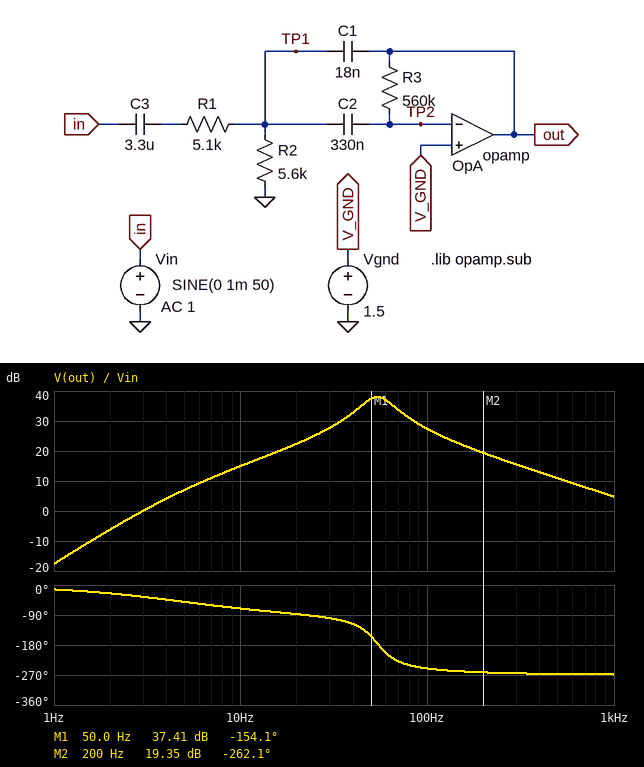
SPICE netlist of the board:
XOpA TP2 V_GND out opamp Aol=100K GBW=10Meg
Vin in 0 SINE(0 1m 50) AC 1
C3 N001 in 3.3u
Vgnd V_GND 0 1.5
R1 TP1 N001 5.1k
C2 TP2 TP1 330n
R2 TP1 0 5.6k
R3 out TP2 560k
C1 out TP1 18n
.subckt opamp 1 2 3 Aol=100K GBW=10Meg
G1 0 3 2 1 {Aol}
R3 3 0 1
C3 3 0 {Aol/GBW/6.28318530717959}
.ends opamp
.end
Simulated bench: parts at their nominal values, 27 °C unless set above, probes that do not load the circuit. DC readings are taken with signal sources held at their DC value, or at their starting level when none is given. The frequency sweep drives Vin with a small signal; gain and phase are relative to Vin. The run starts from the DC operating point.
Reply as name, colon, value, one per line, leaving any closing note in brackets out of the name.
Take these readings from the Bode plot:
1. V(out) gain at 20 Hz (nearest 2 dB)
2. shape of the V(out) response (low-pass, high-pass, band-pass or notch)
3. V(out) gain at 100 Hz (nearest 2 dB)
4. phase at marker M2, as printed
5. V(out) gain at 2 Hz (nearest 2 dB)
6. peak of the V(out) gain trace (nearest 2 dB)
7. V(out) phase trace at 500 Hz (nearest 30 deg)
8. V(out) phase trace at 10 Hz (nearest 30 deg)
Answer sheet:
V(out) gain at 20 Hz: 22 dB
shape of the V(out) response: band-pass
V(out) gain at 100 Hz: 28 dB
phase at marker M2, as printed: -262.1 deg
V(out) gain at 2 Hz: -6 dB
peak of the V(out) gain trace: 38 dB
V(out) phase trace at 500 Hz: -270 deg
V(out) phase trace at 10 Hz: -60 deg
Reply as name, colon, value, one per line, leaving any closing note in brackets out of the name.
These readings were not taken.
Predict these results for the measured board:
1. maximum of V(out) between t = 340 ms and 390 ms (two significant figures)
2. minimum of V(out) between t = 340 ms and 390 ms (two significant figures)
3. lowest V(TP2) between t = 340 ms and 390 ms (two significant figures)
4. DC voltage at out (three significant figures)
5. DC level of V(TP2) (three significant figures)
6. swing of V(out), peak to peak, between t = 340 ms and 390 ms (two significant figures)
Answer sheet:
maximum of V(out) between t = 340 ms and 390 ms: 1.6 V
minimum of V(out) between t = 340 ms and 390 ms: 1.4 V
lowest V(TP2) between t = 340 ms and 390 ms: 1.5 V
DC voltage at out: 1.50 V
DC level of V(TP2): 1.50 V
swing of V(out), peak to peak, between t = 340 ms and 390 ms: 150 mV
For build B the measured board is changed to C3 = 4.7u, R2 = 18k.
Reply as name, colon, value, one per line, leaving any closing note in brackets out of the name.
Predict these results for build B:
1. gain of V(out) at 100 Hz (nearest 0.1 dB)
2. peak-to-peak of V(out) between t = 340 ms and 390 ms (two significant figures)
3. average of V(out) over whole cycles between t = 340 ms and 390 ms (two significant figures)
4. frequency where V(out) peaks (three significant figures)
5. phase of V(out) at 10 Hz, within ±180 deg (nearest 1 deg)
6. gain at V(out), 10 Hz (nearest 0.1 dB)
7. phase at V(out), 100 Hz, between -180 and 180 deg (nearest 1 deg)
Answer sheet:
gain of V(out) at 100 Hz: 26.4 dB
peak-to-peak of V(out) between t = 340 ms and 390 ms: 140 mV
average of V(out) over whole cycles between t = 340 ms and 390 ms: 1.5 V
frequency where V(out) peaks: 44.7 Hz
phase of V(out) at 10 Hz, within ±180 deg: -89 deg
gain at V(out), 10 Hz: 19.1 dB
phase at V(out), 100 Hz, between -180 and 180 deg: 106 deg
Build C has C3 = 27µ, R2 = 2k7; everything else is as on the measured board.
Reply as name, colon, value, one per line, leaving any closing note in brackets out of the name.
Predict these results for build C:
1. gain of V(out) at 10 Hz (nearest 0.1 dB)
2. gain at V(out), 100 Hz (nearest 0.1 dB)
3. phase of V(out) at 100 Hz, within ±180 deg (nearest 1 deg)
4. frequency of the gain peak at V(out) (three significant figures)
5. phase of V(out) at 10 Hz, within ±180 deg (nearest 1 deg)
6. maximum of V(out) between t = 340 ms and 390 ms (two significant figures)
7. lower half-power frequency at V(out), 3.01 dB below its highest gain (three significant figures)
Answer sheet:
gain of V(out) at 10 Hz: 12.2 dB
gain at V(out), 100 Hz: 29.3 dB
phase of V(out) at 100 Hz, within ±180 deg: 107 deg
frequency of the gain peak at V(out): 65.7 Hz
phase of V(out) at 10 Hz, within ±180 deg: -88 deg
maximum of V(out) between t = 340 ms and 390 ms: 1.5 V
lower half-power frequency at V(out), 3.01 dB below its highest gain: 57.7 Hz
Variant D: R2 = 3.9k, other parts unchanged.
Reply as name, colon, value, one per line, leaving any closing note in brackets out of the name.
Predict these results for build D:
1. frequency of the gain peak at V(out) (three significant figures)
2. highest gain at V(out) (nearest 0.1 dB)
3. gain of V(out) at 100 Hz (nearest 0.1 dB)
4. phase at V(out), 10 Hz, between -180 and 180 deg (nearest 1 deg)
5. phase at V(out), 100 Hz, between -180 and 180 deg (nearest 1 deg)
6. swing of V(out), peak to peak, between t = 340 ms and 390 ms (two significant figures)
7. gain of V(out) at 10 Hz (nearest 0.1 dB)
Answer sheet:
frequency of the gain peak at V(out): 59.1 Hz
highest gain at V(out): 38.4 dB
gain of V(out) at 100 Hz: 28.1 dB
phase at V(out), 10 Hz, between -180 and 180 deg: -66 deg
phase at V(out), 100 Hz, between -180 and 180 deg: 111 deg
swing of V(out), peak to peak, between t = 340 ms and 390 ms: 120 mV
gain of V(out) at 10 Hz: 13.1 dB
